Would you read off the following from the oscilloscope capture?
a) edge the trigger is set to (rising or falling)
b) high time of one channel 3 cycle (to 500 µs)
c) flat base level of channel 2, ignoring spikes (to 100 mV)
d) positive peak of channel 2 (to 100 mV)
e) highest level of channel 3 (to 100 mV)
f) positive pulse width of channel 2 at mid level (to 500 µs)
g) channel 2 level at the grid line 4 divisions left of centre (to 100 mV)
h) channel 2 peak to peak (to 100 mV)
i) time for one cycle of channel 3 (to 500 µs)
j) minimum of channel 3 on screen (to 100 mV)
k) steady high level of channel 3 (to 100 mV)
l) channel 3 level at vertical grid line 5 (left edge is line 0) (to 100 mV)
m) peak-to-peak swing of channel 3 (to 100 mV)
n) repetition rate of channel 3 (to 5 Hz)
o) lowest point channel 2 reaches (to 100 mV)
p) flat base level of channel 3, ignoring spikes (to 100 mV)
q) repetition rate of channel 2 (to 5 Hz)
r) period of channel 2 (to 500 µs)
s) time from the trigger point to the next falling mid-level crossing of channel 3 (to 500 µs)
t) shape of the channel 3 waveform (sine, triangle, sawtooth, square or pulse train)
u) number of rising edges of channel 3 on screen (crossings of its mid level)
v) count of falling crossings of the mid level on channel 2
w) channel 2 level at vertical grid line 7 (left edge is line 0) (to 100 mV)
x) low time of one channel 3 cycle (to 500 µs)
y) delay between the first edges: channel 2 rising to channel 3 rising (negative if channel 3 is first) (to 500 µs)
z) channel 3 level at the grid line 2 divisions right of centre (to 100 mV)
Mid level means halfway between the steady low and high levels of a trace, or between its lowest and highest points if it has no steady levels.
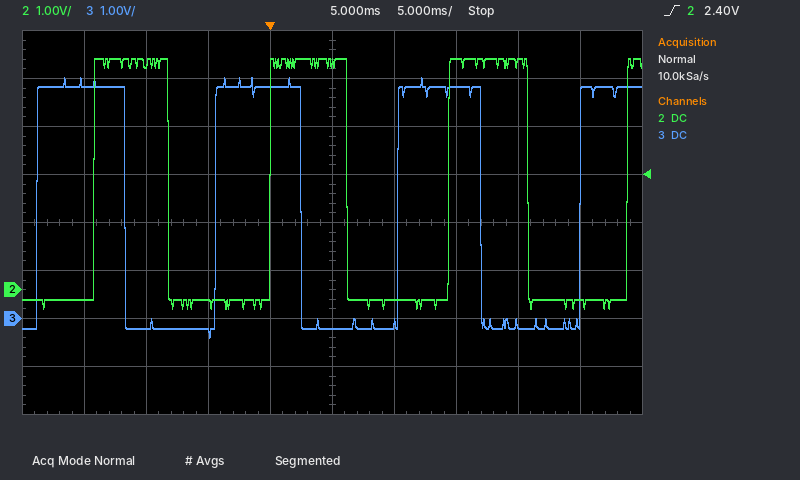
rising
7.0 ms
-200 mV
4.8 V
5.0 V
6.0 ms
-200 mV
5.2 V
14.5 ms
-400 mV
4.8 V
-200 mV
5.4 V
70 Hz
-400 mV
-200 mV
70 Hz
14.5 ms
2.5 ms
square
4
3
4.8 V
7.5 ms
-4.5 ms
4.8 V
